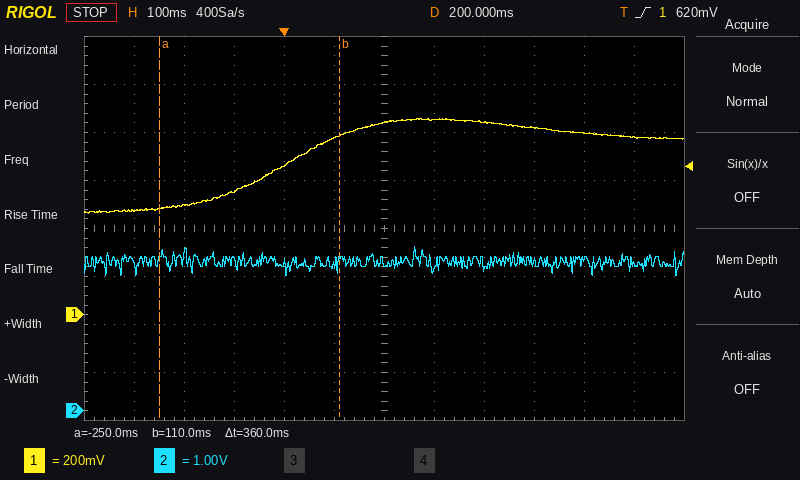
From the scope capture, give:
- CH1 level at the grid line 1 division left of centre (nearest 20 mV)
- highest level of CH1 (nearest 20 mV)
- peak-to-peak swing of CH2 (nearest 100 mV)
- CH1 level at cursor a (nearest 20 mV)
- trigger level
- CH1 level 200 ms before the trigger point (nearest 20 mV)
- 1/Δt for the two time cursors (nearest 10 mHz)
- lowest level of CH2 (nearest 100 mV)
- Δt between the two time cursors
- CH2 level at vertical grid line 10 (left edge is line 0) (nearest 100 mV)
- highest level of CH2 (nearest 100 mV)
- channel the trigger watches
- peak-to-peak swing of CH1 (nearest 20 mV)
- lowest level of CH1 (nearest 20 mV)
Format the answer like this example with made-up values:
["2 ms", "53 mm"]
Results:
["740 mV", "820 mV", "600 mV", "440 mV", "620 mV", "460 mV", "2.78 Hz", "2.8 V", "360 ms", "3.1 V", "3.4 V", "CH1", "400 mV", "420 mV"]
